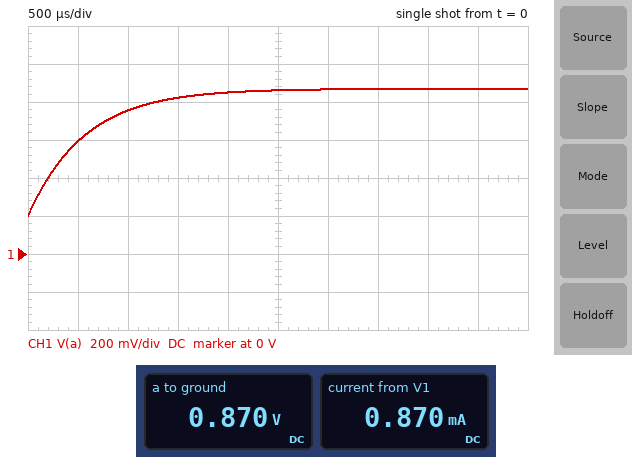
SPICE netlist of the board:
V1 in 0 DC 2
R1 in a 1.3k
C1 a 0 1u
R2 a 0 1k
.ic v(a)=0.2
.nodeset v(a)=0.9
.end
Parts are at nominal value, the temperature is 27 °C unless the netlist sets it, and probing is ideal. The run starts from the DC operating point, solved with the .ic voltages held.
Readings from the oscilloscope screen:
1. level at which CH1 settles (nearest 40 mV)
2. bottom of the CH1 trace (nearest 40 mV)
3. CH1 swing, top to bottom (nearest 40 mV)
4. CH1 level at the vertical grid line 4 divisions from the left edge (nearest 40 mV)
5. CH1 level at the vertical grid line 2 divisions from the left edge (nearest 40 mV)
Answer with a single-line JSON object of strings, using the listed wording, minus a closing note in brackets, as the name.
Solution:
{"level at which CH1 settles": "880 mV", "bottom of the CH1 trace": "200 mV", "CH1 swing, top to bottom": "680 mV", "CH1 level at the vertical grid line 4 divisions from the left edge": "840 mV", "CH1 level at the vertical grid line 2 divisions from the left edge": "760 mV"}
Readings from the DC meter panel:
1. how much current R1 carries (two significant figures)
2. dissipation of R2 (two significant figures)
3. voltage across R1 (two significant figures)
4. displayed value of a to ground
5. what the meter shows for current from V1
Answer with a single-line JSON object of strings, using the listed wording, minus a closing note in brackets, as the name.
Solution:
{"how much current R1 carries": "870 µA", "dissipation of R2": "760 µW", "voltage across R1": "1.1 V", "displayed value of a to ground": "0.870 V", "what the meter shows for current from V1": "0.870 mA"}
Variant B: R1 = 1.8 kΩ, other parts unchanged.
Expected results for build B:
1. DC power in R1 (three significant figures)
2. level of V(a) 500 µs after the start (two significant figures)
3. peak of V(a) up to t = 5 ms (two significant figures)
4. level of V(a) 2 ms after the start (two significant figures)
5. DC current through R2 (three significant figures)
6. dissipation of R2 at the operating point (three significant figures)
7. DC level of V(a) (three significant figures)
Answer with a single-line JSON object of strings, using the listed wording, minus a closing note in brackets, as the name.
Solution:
{"DC power in R1": "918 µW", "level of V(a) 500 µs after the start": "480 mV", "peak of V(a) up to t = 5 ms": "710 mV", "level of V(a) 2 ms after the start": "690 mV", "DC current through R2": "714 µA", "dissipation of R2 at the operating point": "510 µW", "DC level of V(a)": "714 mV"}
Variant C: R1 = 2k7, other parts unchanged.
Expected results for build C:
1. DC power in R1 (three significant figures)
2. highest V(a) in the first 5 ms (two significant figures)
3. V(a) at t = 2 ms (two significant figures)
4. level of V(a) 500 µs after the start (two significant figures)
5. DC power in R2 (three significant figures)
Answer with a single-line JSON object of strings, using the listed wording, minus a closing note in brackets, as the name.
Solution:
{"DC power in R1": "789 µW", "highest V(a) in the first 5 ms": "540 mV", "V(a) at t = 2 ms": "520 mV", "level of V(a) 500 µs after the start": "370 mV", "DC power in R2": "292 µW"}
